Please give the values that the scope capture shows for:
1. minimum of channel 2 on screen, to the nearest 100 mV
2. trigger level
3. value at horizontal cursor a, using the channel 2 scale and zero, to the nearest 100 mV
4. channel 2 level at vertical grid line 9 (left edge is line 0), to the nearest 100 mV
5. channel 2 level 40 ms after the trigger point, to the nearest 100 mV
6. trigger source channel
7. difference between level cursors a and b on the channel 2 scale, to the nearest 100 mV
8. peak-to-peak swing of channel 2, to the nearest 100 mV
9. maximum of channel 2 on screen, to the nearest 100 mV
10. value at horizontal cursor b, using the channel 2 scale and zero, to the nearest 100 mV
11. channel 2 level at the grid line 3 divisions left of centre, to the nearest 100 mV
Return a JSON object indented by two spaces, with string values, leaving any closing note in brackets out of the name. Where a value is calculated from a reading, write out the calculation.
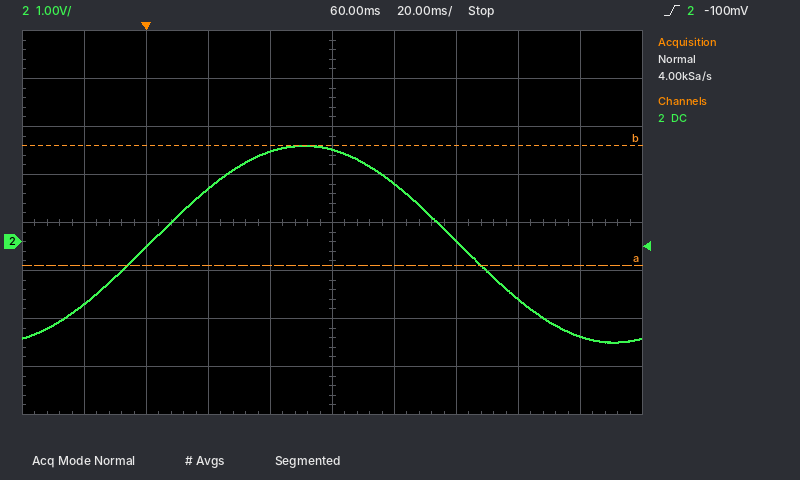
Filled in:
{
  "minimum of channel 2 on screen, to the nearest 100 mV": "-2.1 V",
  "trigger level": "-100 mV",
  "value at horizontal cursor a, using the channel 2 scale and zero, to the nearest 100 mV": "-500 mV",
  "channel 2 level at vertical grid line 9 (left edge is line 0), to the nearest 100 mV": "-2.0 V",
  "channel 2 level 40 ms after the trigger point, to the nearest 100 mV": "1.9 V",
  "trigger source channel": "channel 2",
  "difference between level cursors a and b on the channel 2 scale, to the nearest 100 mV": "2.5 V",
  "peak-to-peak swing of channel 2, to the nearest 100 mV": "2.0 V − (-2.1 V) = 4.1 V",
  "maximum of channel 2 on screen, to the nearest 100 mV": "2.0 V",
  "value at horizontal cursor b, using the channel 2 scale and zero, to the nearest 100 mV": "2.0 V",
  "channel 2 level at the grid line 3 divisions left of centre, to the nearest 100 mV": "-100 mV"
}
